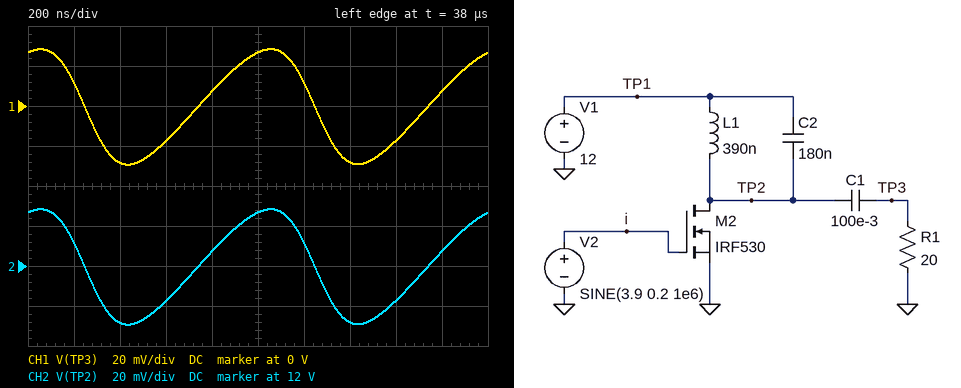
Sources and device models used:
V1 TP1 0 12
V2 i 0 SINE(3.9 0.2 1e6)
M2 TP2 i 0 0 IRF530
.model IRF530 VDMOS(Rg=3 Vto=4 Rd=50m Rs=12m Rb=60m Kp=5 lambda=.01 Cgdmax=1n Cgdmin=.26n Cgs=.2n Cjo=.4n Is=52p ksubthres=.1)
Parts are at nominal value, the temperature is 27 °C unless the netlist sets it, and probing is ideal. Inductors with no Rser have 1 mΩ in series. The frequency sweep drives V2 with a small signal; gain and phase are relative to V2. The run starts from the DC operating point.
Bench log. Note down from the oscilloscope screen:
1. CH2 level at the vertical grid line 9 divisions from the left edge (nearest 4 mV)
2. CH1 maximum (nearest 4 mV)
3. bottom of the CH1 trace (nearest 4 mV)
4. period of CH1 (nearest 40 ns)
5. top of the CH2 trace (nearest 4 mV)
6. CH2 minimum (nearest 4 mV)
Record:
12.008 V
28 mV
-28 mV
1.00 µs
12.028 V
11.972 V
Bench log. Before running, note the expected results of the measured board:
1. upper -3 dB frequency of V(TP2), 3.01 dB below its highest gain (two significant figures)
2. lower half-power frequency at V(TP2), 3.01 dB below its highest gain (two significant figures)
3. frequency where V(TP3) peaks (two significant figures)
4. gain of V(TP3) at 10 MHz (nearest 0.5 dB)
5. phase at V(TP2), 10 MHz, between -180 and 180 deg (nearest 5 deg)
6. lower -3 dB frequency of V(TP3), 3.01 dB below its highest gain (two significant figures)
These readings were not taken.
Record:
620 kHz
580 kHz
600 kHz
-47.0 dB
65 deg
580 kHz
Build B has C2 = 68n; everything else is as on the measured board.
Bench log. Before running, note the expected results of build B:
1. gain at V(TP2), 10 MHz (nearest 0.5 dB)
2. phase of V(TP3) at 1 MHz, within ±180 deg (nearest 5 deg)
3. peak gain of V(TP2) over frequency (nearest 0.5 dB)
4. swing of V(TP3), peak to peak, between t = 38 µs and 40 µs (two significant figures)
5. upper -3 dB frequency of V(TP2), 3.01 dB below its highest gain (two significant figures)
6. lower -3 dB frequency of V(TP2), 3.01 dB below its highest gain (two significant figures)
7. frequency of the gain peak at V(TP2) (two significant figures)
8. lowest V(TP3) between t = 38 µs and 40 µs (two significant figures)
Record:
-38.5 dB
155 deg
-0.5 dB
740 mV
1.0 MHz
920 kHz
970 kHz
-380 mV
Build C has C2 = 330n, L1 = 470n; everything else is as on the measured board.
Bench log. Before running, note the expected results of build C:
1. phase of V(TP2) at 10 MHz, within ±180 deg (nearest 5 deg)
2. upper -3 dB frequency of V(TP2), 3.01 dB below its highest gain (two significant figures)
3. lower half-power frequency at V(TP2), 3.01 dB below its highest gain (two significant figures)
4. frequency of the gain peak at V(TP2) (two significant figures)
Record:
65 deg
420 kHz
390 kHz
400 kHz
